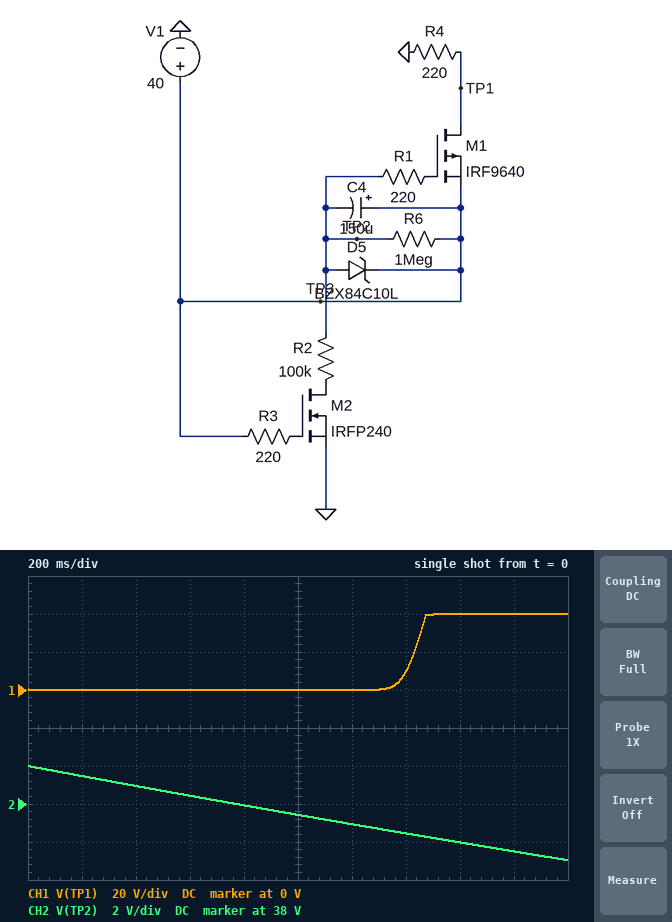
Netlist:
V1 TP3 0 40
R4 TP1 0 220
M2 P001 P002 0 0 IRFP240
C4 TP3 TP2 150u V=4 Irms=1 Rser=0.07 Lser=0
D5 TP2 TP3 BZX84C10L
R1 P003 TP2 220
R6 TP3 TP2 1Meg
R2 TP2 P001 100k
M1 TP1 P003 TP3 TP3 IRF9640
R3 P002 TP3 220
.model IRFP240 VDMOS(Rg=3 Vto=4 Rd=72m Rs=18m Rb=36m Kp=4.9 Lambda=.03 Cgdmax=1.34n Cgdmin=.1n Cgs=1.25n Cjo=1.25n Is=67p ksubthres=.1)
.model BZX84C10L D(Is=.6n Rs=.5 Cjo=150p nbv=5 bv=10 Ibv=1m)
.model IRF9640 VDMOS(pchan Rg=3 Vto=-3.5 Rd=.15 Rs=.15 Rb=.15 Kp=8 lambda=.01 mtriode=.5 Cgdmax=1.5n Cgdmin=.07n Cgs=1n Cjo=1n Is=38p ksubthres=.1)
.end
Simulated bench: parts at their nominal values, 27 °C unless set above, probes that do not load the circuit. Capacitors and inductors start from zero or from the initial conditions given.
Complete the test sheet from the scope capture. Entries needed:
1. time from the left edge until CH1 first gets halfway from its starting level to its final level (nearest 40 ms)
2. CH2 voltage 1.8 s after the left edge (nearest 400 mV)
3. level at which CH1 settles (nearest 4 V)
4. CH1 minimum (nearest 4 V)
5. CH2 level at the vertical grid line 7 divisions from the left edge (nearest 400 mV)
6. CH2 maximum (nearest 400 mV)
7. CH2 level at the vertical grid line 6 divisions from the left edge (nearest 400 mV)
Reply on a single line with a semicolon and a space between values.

1.44 s; 35.6 V; 40 V; 0 V; 36.4 V; 40.0 V; 36.8 V
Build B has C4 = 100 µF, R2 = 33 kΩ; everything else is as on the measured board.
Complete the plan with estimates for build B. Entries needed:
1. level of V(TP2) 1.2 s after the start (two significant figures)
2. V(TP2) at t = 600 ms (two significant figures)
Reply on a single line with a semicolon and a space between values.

30 V; 33 V
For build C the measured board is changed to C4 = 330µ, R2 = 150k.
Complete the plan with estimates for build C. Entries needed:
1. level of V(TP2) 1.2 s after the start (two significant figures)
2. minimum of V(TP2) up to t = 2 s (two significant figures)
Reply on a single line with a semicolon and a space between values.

39 V; 38 V
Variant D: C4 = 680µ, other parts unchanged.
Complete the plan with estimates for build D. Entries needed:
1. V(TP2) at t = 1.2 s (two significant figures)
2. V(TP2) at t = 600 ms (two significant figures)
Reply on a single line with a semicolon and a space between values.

39 V; 40 V
